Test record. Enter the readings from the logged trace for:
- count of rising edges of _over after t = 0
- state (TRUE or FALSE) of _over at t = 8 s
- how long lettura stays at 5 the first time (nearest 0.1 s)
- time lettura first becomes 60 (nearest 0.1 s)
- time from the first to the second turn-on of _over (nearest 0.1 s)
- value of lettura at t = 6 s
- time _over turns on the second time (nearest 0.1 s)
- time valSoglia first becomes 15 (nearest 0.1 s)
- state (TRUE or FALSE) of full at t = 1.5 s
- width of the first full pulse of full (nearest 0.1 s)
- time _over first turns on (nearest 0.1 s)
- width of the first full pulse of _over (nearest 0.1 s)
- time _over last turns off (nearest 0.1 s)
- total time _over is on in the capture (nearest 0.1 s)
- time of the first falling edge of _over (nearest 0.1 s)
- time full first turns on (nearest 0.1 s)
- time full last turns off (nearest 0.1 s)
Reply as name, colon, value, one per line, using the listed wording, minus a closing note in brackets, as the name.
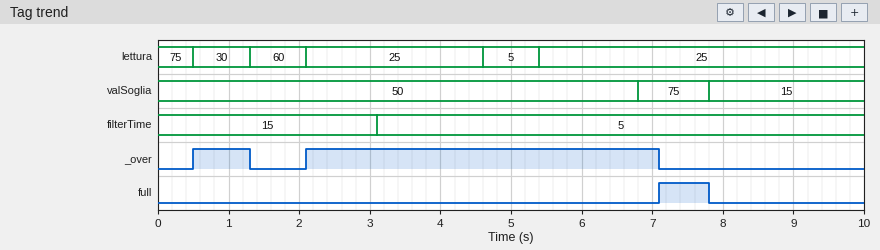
count of rising edges of _over after t = 0: 2
state (TRUE or FALSE) of _over at t = 8 s: FALSE
how long lettura stays at 5 the first time: 0.8 s
time lettura first becomes 60: 1.3 s
time from the first to the second turn-on of _over: 1.6 s
value of lettura at t = 6 s: 25
time _over turns on the second time: 2.1 s
time valSoglia first becomes 15: 7.8 s
state (TRUE or FALSE) of full at t = 1.5 s: FALSE
width of the first full pulse of full: 0.7 s
time _over first turns on: 0.5 s
width of the first full pulse of _over: 0.8 s
time _over last turns off: 7.1 s
total time _over is on in the capture: 5.8 s
time of the first falling edge of _over: 1.3 s
time full first turns on: 7.1 s
time full last turns off: 7.8 s
